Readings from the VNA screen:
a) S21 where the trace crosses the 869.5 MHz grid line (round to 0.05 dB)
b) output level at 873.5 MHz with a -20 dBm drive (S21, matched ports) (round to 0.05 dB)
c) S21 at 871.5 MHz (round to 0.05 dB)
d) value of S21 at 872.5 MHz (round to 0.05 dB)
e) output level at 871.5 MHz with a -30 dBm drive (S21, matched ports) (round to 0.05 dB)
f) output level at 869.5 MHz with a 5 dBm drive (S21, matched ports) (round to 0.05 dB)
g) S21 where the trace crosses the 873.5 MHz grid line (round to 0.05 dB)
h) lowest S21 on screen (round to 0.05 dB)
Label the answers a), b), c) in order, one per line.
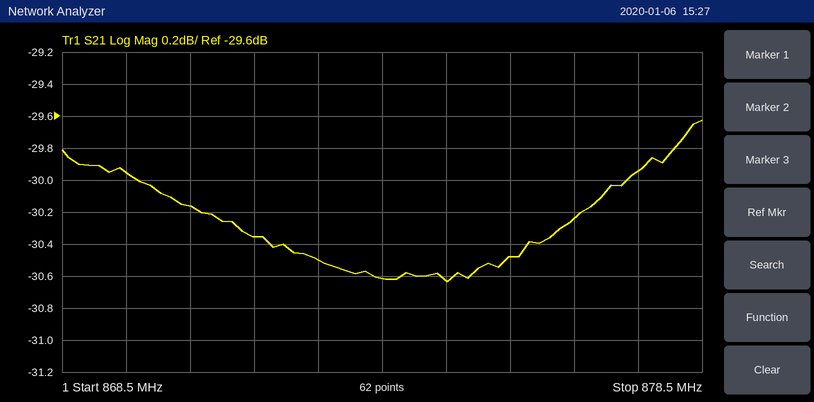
a) -29.95 dB
b) -50.60 dBm
c) -30.35 dB
d) -30.50 dB
e) -60.35 dBm
f) -24.95 dBm
g) -30.60 dB
h) -30.65 dB
